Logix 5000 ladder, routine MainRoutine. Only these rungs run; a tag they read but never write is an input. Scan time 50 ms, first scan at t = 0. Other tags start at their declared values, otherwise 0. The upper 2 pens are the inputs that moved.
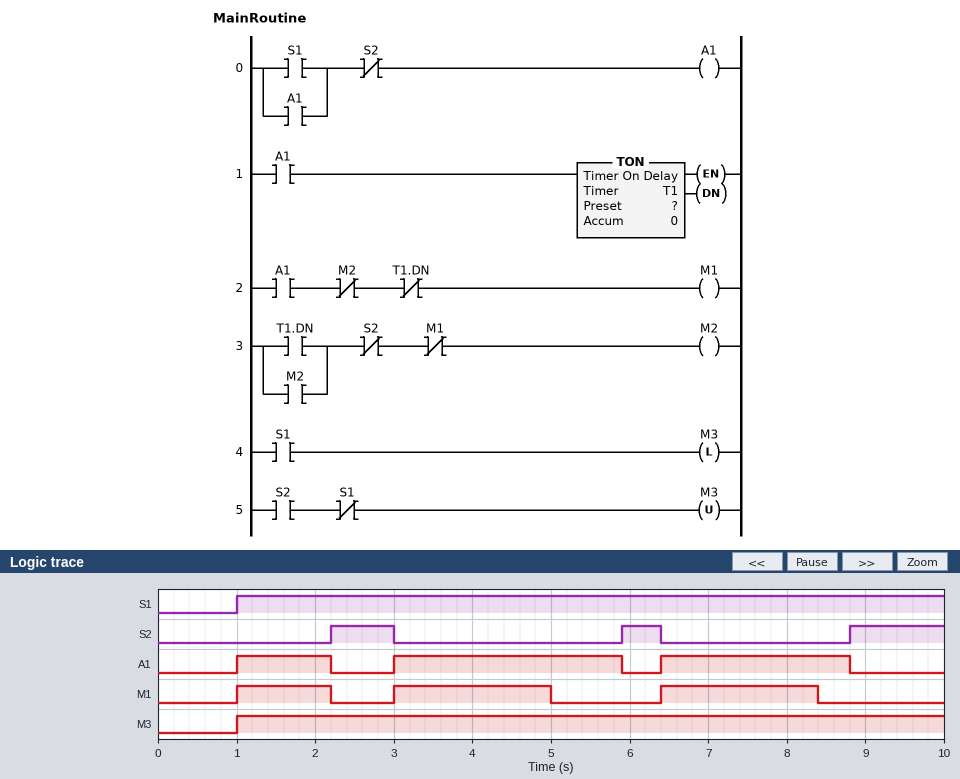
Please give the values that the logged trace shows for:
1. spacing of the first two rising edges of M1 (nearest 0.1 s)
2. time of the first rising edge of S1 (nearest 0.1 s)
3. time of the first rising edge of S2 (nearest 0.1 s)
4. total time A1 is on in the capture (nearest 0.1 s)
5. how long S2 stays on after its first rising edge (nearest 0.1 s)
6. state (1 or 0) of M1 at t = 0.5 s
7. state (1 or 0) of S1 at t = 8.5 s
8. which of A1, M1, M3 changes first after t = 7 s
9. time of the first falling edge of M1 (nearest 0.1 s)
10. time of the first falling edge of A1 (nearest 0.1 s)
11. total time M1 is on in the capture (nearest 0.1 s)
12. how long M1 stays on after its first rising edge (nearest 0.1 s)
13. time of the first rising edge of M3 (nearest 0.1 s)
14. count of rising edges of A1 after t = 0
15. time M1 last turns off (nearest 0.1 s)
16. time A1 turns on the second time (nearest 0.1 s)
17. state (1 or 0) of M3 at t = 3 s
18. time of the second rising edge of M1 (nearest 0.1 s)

2.0 s
1.0 s
2.2 s
6.5 s
0.8 s
0
1
M1
2.2 s
2.2 s
5.2 s
1.2 s
1.0 s
3
8.4 s
3.0 s
1
3.0 s
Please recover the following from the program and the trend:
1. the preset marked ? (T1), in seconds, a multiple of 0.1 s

2.0 s
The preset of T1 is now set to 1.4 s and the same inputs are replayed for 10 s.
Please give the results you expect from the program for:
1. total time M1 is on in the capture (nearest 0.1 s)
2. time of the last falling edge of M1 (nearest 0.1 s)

4.0 s
7.8 s
